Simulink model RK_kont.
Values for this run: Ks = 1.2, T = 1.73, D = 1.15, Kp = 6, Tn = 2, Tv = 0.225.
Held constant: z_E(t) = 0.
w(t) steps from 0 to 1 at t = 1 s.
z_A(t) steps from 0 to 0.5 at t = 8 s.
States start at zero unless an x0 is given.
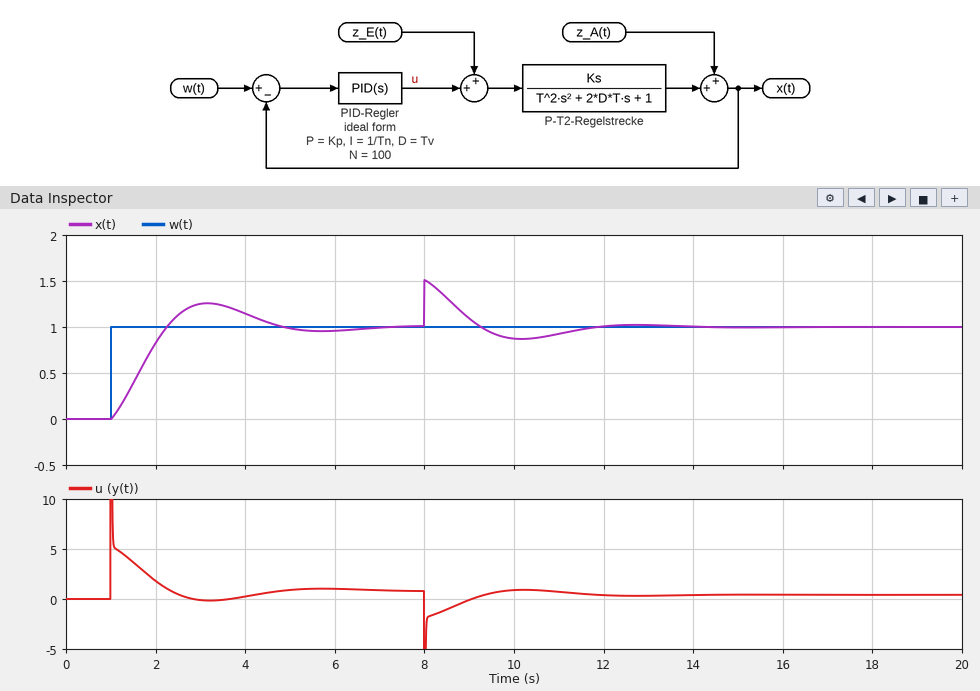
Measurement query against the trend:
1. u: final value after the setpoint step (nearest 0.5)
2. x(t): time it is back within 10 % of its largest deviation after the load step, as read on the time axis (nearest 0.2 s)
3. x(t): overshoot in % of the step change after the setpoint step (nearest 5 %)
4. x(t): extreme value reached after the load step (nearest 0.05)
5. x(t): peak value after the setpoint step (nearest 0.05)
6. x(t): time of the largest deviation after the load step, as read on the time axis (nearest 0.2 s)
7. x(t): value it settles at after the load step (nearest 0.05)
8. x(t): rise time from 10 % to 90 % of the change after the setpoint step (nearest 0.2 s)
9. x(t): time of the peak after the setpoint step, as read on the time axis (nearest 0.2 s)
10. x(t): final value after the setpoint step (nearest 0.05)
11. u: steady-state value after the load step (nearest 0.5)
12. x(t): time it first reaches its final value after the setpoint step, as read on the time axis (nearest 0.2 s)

1.0
11.2 s
25 %
1.50
1.25
8.0 s
1.00
1.0 s
3.2 s
1.00
0.5
2.2 s
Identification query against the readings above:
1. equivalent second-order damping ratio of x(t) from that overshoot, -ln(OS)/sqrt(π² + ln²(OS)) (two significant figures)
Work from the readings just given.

0.40
